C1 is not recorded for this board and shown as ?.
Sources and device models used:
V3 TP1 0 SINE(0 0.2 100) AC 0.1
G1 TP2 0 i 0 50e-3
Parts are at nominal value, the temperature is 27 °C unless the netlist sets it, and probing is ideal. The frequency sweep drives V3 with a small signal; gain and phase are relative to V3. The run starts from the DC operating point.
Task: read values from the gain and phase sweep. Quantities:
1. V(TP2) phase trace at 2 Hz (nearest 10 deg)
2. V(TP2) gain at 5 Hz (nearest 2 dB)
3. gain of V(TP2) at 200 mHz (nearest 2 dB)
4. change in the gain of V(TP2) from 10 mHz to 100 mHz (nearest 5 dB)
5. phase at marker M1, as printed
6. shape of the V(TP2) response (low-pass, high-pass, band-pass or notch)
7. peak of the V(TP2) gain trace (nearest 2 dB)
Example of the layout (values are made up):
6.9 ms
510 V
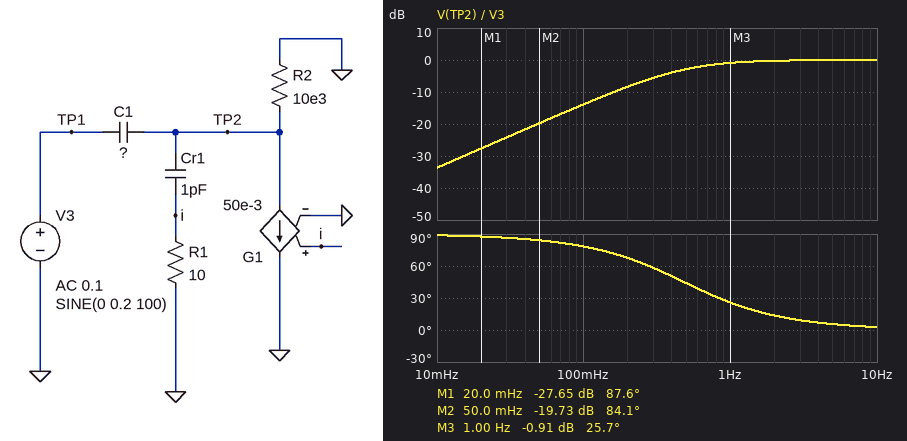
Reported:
10 deg
0 dB
-8 dB
20 dB
87.6 deg
high-pass
0 dB
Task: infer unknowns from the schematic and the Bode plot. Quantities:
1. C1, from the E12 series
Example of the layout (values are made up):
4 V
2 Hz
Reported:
33 µF
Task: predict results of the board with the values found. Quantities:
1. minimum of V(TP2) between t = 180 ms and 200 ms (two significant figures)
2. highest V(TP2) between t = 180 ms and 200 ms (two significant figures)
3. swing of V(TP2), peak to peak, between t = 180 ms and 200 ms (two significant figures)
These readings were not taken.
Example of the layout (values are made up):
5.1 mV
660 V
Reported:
-200 mV
200 mV
400 mV
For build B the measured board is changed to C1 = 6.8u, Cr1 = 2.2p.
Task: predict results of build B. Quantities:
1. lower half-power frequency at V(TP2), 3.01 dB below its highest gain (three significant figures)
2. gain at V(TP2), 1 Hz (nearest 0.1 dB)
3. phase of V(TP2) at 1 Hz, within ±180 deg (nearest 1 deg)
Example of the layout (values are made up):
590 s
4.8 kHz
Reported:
2.34 Hz
-8.1 dB
67 deg
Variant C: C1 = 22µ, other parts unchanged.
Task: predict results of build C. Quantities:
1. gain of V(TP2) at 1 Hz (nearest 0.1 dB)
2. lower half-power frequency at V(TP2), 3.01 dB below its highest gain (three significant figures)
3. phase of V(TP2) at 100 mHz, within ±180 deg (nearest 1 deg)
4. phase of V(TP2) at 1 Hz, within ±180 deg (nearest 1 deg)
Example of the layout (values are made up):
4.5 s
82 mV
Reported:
-1.8 dB
723 mHz
82 deg
36 deg
